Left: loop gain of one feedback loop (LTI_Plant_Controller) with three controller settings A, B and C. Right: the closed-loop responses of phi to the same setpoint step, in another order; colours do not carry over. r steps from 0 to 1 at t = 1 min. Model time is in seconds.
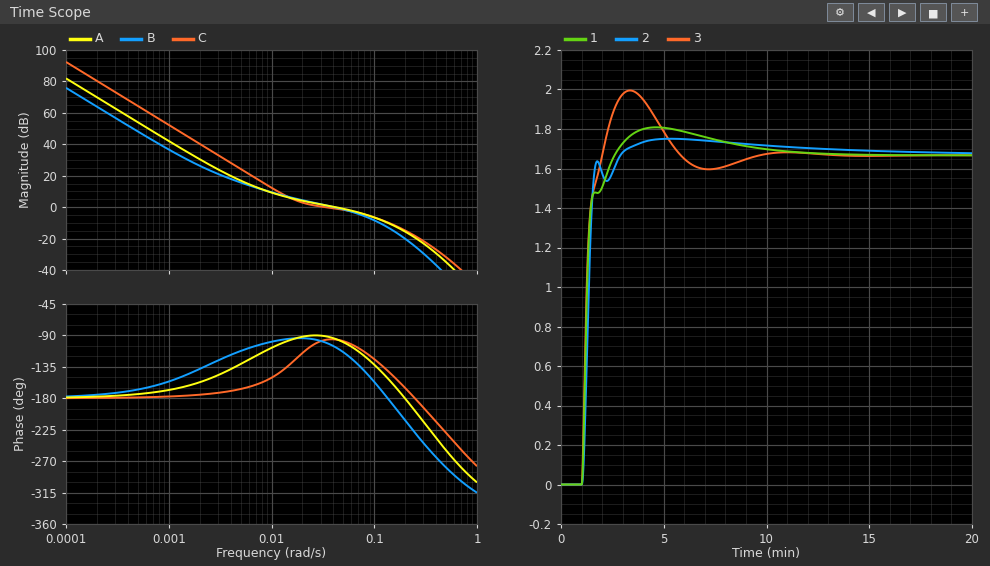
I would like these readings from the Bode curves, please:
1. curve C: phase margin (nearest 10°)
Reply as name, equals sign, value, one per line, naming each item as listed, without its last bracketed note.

curve C: phase margin = 80°
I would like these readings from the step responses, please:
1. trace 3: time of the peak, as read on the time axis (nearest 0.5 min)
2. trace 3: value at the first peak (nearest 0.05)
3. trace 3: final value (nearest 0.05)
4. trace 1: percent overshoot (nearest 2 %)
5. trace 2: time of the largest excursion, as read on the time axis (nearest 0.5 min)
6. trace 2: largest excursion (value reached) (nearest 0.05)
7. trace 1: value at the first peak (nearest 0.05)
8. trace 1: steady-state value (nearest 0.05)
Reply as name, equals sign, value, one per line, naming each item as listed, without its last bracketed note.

trace 3: time of the peak, as read on the time axis = 3.5 min
trace 3: value at the first peak = 2.00
trace 3: final value = 1.65
trace 1: percent overshoot = 8 %
trace 2: time of the largest excursion, as read on the time axis = 5.5 min
trace 2: largest excursion (value reached) = 1.75
trace 1: value at the first peak = 1.80
trace 1: steady-state value = 1.65
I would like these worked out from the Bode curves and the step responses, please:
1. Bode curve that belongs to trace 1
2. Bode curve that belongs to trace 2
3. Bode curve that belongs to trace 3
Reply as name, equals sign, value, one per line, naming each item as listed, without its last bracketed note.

Bode curve that belongs to trace 1 = A
Bode curve that belongs to trace 2 = B
Bode curve that belongs to trace 3 = C
